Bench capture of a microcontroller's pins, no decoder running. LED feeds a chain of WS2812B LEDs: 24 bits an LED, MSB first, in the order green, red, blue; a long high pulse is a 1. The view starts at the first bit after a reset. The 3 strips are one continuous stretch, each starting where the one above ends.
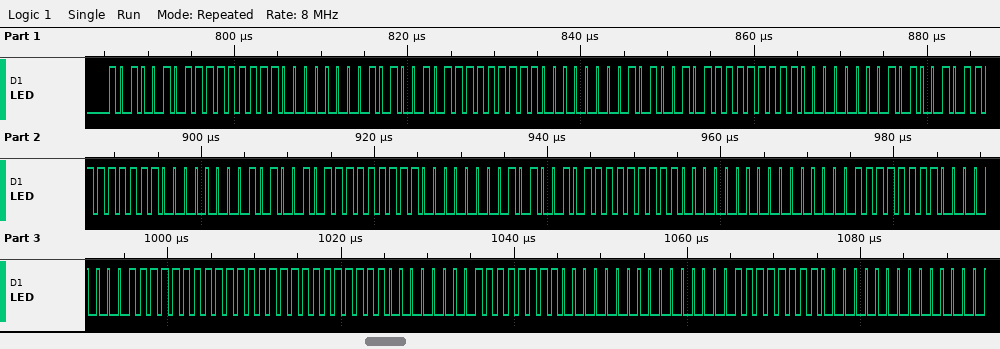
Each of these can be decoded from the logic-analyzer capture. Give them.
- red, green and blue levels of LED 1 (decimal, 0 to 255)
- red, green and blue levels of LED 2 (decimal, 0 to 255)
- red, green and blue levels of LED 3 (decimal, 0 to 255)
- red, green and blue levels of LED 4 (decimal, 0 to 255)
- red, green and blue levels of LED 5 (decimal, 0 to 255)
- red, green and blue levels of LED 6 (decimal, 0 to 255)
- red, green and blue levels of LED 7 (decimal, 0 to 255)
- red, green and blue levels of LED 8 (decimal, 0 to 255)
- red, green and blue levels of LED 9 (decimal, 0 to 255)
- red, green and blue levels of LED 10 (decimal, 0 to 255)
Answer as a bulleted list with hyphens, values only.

- 255, 165, 0
- 255, 165, 0
- 255, 165, 0
- 255, 165, 0
- 255, 165, 0
- 255, 165, 0
- 255, 0, 0
- 255, 255, 255
- 255, 0, 0
- 255, 0, 0
